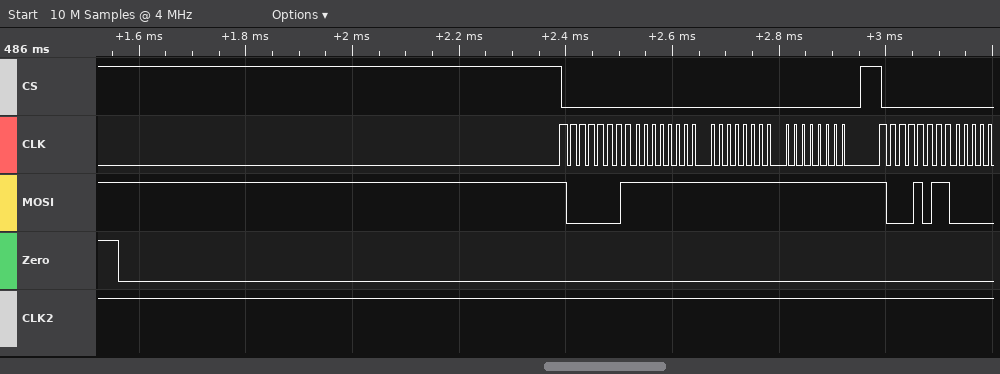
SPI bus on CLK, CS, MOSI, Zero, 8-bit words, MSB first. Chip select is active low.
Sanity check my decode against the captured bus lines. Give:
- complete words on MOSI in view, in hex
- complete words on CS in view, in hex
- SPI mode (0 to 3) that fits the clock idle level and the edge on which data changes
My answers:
81, FF, FF, FF, 8B
80, 00, 00, 00, 80
0
